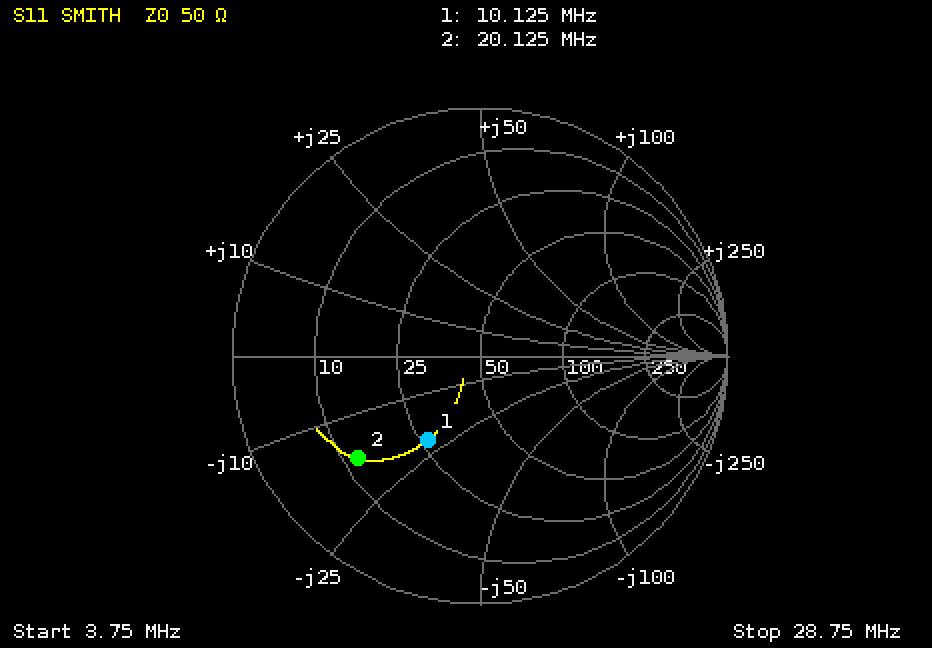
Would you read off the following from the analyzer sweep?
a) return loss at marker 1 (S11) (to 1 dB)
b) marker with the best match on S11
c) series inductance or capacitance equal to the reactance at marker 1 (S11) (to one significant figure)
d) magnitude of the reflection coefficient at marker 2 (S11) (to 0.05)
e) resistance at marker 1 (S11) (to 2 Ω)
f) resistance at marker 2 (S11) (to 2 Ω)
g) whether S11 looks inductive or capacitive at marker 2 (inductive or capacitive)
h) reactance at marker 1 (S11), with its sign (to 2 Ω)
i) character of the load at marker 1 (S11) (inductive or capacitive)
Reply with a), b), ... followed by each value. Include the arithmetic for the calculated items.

a) 8 dB
b) marker 1
c) C = 1/(2π × 10.125 MHz × 22 Ω) ≈ 715 pF, so 700 pF to one significant figure
d) 0.65
e) 26 Ω
f) 12 Ω
g) capacitive
h) -22 Ω
i) capacitive
